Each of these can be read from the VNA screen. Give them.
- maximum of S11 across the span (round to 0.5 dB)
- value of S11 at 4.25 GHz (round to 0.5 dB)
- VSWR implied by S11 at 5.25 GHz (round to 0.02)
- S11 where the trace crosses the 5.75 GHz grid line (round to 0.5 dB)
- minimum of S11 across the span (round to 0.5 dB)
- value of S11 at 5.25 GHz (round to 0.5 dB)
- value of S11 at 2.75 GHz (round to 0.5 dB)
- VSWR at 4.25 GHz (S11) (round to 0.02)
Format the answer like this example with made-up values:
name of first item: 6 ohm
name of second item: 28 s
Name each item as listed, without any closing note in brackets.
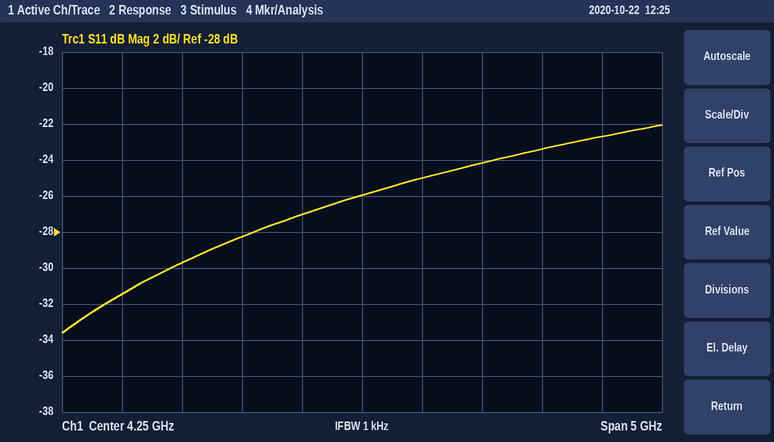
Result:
maximum of S11 across the span: -22.0 dB
value of S11 at 4.25 GHz: -26.0 dB
VSWR implied by S11 at 5.25 GHz: 1.14
S11 where the trace crosses the 5.75 GHz grid line: -23.5 dB
minimum of S11 across the span: -33.5 dB
value of S11 at 5.25 GHz: -24.0 dB
value of S11 at 2.75 GHz: -29.5 dB
VSWR at 4.25 GHz (S11): 1.10
